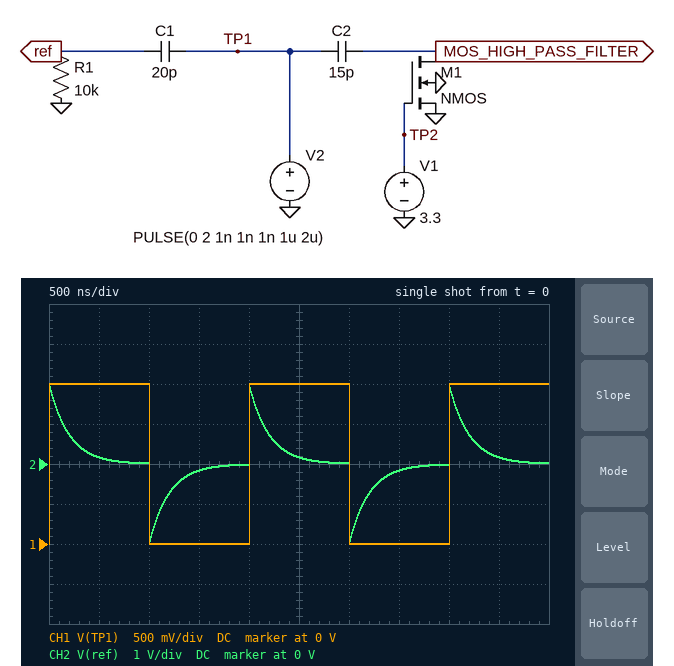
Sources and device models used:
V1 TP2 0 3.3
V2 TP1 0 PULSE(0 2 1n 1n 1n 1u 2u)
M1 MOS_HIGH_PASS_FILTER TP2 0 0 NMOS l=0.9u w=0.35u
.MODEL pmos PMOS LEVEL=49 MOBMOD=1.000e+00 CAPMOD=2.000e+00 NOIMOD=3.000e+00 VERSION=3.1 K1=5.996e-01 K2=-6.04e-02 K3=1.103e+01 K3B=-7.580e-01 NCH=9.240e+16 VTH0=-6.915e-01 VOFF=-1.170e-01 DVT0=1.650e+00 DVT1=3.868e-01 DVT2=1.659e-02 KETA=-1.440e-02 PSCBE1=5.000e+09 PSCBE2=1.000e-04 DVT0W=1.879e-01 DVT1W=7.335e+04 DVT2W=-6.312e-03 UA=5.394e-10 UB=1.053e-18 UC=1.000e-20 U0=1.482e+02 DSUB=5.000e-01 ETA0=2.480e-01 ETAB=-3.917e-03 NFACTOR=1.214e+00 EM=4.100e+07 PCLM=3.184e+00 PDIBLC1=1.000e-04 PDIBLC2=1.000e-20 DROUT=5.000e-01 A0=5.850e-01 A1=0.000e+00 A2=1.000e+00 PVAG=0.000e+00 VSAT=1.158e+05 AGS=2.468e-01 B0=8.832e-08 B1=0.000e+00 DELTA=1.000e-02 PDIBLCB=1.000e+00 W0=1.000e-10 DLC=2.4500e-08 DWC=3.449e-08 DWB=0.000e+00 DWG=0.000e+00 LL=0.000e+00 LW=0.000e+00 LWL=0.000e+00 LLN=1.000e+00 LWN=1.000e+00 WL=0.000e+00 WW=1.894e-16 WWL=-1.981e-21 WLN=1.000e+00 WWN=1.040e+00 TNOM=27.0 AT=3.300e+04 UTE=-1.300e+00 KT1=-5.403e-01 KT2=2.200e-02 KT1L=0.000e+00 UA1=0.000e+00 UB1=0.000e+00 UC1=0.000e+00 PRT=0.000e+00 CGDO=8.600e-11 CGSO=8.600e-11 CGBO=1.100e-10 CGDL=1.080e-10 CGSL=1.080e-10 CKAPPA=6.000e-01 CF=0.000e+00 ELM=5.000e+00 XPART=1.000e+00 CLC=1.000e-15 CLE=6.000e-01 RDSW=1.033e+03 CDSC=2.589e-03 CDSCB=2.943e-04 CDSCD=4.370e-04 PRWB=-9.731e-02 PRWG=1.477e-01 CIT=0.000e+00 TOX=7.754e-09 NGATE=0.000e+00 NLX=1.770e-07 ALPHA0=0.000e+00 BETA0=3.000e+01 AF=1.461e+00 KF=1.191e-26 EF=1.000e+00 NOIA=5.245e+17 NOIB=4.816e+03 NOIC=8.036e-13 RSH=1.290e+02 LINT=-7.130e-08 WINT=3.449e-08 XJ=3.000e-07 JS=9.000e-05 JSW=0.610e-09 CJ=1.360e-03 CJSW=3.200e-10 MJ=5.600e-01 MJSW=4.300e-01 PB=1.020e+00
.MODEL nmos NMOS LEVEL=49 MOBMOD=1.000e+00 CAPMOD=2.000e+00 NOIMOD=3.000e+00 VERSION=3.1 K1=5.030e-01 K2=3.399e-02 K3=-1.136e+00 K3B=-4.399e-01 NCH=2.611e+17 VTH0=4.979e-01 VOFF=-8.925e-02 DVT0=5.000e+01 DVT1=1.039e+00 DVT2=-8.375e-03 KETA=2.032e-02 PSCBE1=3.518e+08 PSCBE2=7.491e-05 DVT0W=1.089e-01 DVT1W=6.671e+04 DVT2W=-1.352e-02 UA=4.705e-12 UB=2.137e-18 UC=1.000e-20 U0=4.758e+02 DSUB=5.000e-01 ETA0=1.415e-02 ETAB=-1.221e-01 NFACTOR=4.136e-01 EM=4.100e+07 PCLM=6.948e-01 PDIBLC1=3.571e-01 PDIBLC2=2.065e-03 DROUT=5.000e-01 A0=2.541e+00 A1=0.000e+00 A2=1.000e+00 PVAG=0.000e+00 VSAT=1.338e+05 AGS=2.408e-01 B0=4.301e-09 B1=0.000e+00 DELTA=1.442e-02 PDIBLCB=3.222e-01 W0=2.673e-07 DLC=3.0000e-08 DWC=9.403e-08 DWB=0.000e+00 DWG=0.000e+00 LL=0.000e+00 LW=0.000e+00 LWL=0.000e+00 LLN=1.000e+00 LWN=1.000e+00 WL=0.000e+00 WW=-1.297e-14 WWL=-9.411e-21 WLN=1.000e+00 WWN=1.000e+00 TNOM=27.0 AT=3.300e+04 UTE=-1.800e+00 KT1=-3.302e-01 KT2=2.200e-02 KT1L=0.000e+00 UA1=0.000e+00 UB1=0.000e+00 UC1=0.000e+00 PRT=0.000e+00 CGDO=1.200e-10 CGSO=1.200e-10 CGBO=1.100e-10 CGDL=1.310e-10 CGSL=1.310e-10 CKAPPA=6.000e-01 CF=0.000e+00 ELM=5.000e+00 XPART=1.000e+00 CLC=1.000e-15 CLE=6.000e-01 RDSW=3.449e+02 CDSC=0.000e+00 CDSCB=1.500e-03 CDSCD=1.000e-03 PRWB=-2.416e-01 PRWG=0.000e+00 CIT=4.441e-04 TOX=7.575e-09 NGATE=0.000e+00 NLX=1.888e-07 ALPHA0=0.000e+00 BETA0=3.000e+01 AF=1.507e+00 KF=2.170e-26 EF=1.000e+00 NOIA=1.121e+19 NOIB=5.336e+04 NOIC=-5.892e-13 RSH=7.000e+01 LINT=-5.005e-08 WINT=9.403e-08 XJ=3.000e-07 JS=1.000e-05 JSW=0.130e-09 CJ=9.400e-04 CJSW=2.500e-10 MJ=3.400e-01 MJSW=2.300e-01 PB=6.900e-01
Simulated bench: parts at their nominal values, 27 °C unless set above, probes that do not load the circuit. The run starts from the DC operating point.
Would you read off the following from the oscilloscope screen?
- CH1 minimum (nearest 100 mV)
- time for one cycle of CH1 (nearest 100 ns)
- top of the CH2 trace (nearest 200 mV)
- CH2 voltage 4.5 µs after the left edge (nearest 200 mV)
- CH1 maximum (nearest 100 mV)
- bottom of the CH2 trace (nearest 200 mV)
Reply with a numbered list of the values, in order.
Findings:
1. 0 V
2. 2.0 µs
3. 2.0 V
4. 200 mV
5. 2.0 V
6. -2.0 V
